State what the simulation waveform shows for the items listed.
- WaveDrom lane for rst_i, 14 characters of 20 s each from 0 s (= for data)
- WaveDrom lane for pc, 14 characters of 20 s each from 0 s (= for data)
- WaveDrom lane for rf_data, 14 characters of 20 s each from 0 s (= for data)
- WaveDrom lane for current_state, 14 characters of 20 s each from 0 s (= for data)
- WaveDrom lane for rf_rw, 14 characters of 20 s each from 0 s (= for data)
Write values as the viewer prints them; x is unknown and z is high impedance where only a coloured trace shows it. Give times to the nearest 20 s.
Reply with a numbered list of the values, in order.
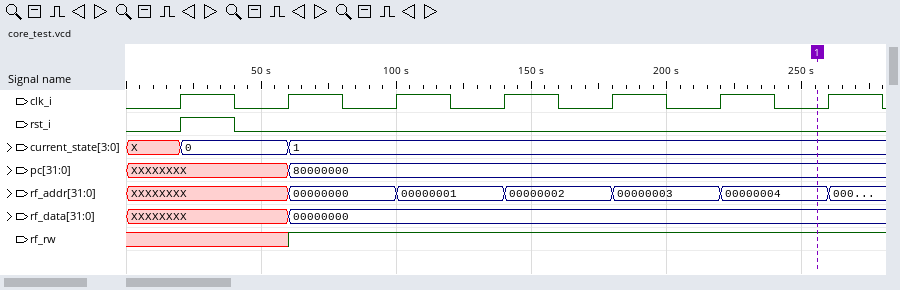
1. {name: 'rst_i', wave: '010...........'}
2. {name: 'pc', wave: 'x..=..........', data: '80000000'}
3. {name: 'rf_data', wave: 'x..=..........', data: '00000000'}
4. {name: 'current_state', wave: 'x=.=..........', data: '0 1'}
5. {name: 'rf_rw', wave: 'x..1..........'}
